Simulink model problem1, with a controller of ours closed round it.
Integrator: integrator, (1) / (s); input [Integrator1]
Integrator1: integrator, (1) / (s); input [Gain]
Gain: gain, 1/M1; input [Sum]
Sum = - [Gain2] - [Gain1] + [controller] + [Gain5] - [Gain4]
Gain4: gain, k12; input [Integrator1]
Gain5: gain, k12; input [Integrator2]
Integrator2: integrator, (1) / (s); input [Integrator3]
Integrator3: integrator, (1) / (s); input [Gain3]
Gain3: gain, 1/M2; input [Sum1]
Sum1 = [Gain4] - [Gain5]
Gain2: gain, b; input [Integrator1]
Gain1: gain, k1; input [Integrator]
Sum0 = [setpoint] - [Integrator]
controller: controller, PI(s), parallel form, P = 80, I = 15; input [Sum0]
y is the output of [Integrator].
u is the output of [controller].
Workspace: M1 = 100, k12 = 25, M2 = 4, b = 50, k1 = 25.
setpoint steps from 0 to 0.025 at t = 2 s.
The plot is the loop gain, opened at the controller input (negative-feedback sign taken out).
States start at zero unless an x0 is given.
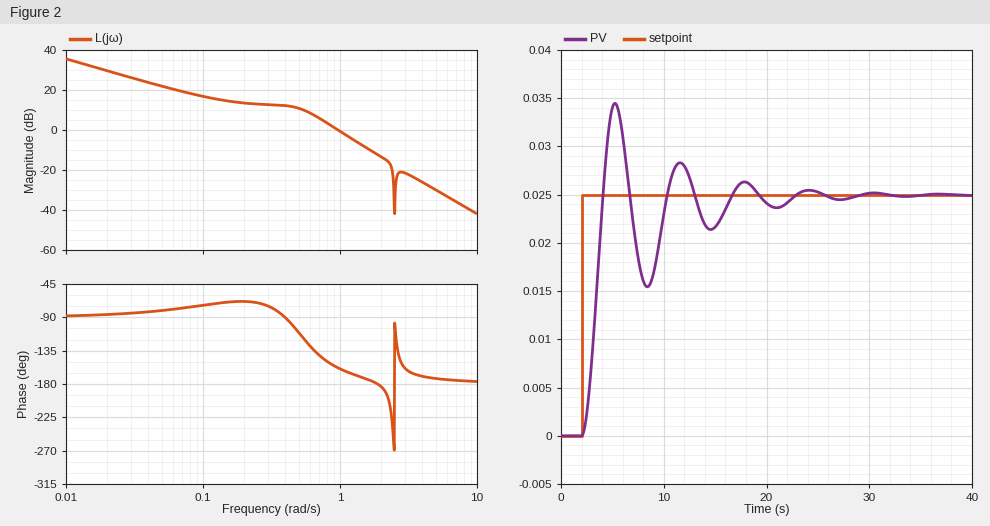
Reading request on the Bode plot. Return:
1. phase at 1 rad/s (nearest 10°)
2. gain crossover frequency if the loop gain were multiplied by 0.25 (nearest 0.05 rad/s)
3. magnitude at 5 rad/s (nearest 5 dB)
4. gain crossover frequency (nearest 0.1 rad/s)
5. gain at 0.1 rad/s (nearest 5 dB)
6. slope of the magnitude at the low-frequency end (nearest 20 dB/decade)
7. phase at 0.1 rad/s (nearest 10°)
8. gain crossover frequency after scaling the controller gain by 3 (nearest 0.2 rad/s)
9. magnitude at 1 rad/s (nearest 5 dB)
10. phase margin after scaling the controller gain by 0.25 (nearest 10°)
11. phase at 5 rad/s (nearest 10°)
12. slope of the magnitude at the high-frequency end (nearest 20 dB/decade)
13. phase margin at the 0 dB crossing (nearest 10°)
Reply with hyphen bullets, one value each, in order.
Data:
- -160°
- 0.40 rad/s
- -30 dB
- 1.0 rad/s
- 15 dB
- -20 dB/decade
- -70°
- 1.6 rad/s
- 0 dB
- 90°
- -170°
- -40 dB/decade
- 20°
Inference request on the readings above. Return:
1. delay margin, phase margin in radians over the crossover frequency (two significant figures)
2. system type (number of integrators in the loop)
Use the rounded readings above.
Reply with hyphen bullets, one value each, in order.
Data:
- 0.35 s
- 1
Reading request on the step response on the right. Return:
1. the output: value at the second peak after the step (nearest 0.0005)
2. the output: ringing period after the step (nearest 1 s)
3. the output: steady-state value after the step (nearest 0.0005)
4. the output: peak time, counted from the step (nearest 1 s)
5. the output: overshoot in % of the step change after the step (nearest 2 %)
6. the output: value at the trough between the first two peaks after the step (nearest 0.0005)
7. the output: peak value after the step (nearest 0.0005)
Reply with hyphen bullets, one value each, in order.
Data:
- 0.0285
- 6 s
- 0.0250
- 3 s
- 38 %
- 0.0155
- 0.0345
